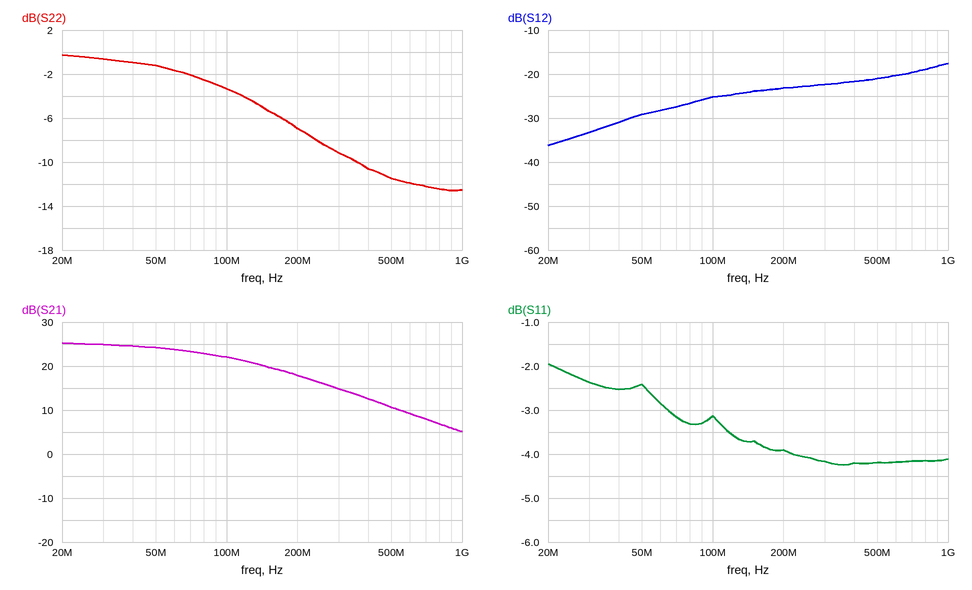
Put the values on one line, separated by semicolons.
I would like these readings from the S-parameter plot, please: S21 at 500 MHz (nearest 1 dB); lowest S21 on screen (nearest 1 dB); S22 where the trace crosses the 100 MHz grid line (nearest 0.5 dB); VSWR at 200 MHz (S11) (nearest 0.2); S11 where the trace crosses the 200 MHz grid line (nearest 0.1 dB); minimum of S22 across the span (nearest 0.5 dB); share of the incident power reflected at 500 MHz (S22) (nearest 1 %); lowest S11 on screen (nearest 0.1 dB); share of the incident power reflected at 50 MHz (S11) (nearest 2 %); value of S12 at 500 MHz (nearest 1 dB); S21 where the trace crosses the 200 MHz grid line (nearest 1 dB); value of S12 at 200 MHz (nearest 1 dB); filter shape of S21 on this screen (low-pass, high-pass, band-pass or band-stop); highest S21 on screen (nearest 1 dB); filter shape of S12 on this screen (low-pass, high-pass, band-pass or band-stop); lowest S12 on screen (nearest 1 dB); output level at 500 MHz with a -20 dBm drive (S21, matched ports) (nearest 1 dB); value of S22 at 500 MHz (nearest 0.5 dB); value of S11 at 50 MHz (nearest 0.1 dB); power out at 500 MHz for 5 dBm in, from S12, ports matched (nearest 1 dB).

11 dB; 5 dB; -3.5 dB; 4.6; -3.9 dB; -12.5 dB; 7 %; -4.2 dB; 58 %; -21 dB; 18 dB; -23 dB; low-pass; 25 dB; high-pass; -36 dB; -9 dBm; -11.5 dB; -2.4 dB; -16 dBm
